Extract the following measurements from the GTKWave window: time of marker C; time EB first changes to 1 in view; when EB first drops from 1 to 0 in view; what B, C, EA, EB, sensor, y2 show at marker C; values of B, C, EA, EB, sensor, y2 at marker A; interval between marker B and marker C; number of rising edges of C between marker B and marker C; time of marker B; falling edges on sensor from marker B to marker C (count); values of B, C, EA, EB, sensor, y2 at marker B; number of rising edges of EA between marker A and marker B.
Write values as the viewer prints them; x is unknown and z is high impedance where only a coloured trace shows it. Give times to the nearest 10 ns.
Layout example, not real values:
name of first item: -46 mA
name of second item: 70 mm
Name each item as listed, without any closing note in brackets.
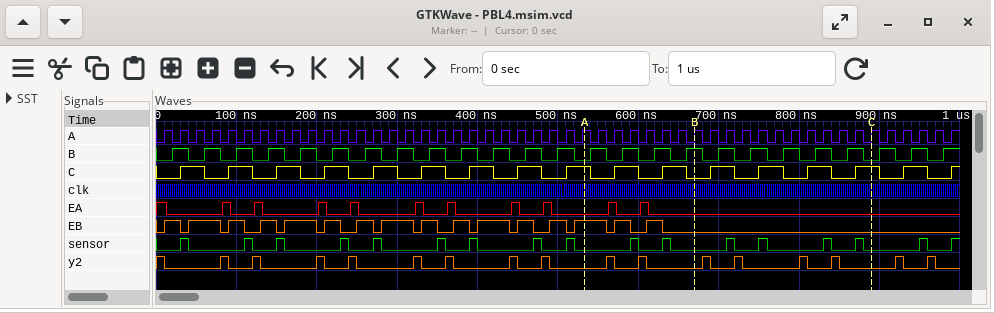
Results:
time of marker C: 890 ns
time EB first changes to 1 in view: 10 ns
when EB first drops from 1 to 0 in view: 30 ns
what B, C, EA, EB, sensor, y2 show at marker C: B=0, C=1, EA=0, EB=0, sensor=0, y2=0
values of B, C, EA, EB, sensor, y2 at marker A: B=0, C=1, EA=0, EB=1, sensor=0, y2=0
interval between marker B and marker C: 220 ns
number of rising edges of C between marker B and marker C: 4
time of marker B: 670 ns
falling edges on sensor from marker B to marker C: 4
values of B, C, EA, EB, sensor, y2 at marker B: B=1, C=0, EA=0, EB=0, sensor=0, y2=0
number of rising edges of EA between marker A and marker B: 2
